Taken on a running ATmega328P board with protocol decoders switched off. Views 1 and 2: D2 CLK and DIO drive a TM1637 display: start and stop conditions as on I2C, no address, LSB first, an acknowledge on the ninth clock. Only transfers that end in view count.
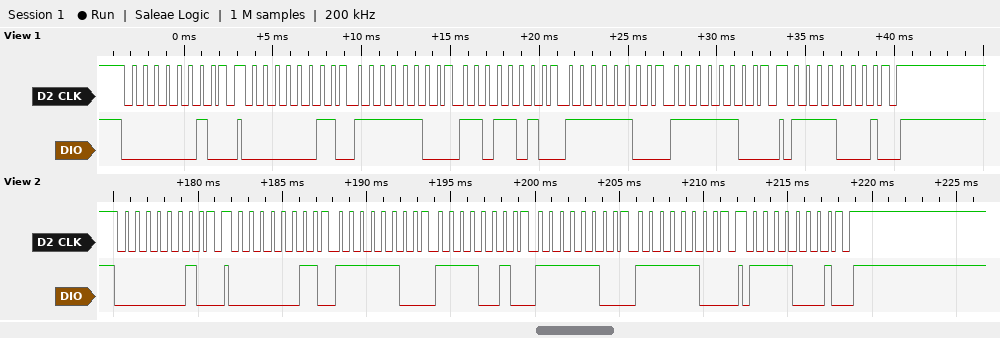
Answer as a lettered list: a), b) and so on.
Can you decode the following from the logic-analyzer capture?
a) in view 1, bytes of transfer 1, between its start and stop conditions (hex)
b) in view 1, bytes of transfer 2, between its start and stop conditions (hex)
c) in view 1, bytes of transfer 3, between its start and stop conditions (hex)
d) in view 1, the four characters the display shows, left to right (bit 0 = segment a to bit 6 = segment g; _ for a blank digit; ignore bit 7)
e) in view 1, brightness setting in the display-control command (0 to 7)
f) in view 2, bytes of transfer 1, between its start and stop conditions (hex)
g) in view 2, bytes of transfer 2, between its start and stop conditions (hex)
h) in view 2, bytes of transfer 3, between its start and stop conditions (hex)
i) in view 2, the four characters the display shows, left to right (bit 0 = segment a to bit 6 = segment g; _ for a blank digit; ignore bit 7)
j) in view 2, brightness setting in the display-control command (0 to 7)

a) 40
b) C0 3F 5B 3F 3F
c) 8F
d) 0200
e) 7
f) 40
g) C0 3F 4F 3F 3F
h) 8F
i) 0300
j) 7
